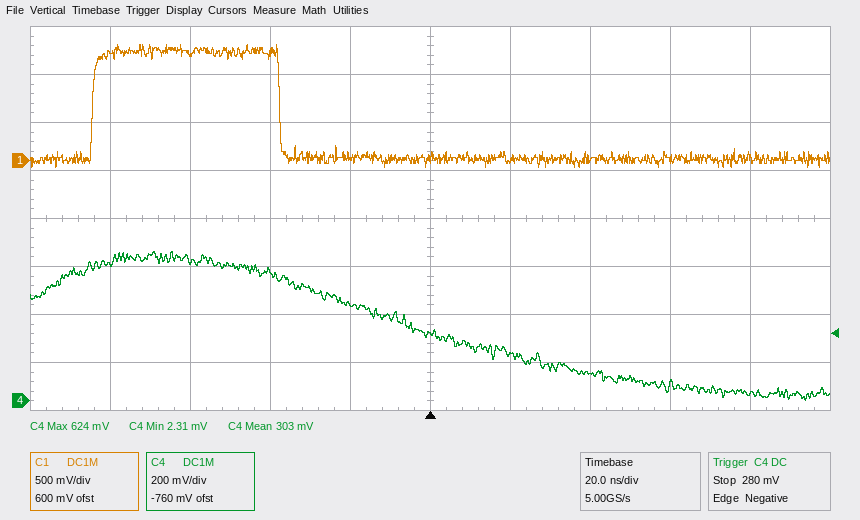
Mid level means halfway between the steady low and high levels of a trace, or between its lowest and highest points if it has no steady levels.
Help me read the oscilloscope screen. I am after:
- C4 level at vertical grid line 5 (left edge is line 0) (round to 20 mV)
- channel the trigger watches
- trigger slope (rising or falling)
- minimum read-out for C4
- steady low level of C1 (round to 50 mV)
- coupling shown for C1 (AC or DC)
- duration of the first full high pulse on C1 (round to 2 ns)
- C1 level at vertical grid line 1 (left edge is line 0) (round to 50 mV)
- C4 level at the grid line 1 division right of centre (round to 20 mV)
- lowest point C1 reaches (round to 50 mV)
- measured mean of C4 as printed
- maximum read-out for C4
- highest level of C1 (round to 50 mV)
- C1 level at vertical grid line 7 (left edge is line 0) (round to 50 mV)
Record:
280 mV
C4
falling
2.31 mV
0 mV
DC
46 ns
1.10 V
200 mV
-50 mV
303 mV
624 mV
1.20 V
0 mV
